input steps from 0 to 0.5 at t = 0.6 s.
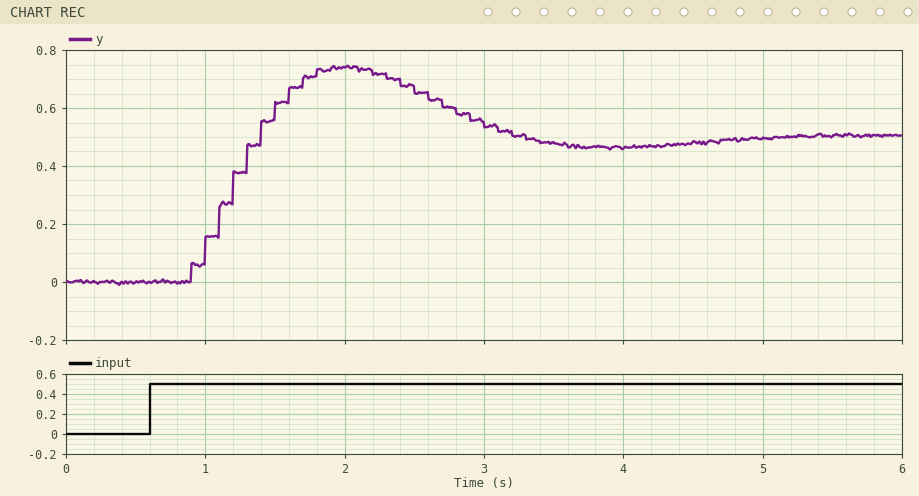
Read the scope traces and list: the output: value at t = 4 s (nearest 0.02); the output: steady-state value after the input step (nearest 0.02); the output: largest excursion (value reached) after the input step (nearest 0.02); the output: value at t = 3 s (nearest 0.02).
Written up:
0.46
0.50
0.74
0.54
